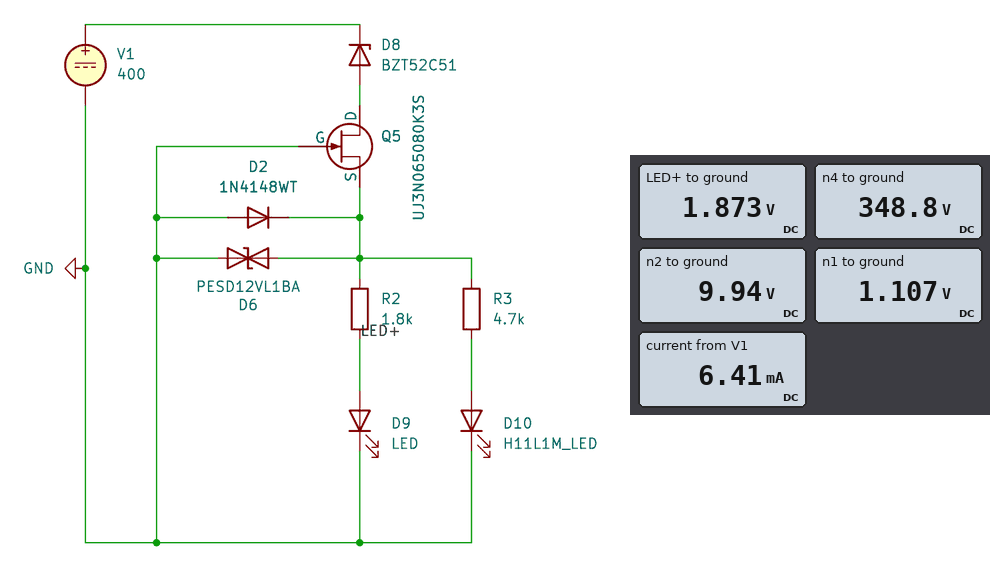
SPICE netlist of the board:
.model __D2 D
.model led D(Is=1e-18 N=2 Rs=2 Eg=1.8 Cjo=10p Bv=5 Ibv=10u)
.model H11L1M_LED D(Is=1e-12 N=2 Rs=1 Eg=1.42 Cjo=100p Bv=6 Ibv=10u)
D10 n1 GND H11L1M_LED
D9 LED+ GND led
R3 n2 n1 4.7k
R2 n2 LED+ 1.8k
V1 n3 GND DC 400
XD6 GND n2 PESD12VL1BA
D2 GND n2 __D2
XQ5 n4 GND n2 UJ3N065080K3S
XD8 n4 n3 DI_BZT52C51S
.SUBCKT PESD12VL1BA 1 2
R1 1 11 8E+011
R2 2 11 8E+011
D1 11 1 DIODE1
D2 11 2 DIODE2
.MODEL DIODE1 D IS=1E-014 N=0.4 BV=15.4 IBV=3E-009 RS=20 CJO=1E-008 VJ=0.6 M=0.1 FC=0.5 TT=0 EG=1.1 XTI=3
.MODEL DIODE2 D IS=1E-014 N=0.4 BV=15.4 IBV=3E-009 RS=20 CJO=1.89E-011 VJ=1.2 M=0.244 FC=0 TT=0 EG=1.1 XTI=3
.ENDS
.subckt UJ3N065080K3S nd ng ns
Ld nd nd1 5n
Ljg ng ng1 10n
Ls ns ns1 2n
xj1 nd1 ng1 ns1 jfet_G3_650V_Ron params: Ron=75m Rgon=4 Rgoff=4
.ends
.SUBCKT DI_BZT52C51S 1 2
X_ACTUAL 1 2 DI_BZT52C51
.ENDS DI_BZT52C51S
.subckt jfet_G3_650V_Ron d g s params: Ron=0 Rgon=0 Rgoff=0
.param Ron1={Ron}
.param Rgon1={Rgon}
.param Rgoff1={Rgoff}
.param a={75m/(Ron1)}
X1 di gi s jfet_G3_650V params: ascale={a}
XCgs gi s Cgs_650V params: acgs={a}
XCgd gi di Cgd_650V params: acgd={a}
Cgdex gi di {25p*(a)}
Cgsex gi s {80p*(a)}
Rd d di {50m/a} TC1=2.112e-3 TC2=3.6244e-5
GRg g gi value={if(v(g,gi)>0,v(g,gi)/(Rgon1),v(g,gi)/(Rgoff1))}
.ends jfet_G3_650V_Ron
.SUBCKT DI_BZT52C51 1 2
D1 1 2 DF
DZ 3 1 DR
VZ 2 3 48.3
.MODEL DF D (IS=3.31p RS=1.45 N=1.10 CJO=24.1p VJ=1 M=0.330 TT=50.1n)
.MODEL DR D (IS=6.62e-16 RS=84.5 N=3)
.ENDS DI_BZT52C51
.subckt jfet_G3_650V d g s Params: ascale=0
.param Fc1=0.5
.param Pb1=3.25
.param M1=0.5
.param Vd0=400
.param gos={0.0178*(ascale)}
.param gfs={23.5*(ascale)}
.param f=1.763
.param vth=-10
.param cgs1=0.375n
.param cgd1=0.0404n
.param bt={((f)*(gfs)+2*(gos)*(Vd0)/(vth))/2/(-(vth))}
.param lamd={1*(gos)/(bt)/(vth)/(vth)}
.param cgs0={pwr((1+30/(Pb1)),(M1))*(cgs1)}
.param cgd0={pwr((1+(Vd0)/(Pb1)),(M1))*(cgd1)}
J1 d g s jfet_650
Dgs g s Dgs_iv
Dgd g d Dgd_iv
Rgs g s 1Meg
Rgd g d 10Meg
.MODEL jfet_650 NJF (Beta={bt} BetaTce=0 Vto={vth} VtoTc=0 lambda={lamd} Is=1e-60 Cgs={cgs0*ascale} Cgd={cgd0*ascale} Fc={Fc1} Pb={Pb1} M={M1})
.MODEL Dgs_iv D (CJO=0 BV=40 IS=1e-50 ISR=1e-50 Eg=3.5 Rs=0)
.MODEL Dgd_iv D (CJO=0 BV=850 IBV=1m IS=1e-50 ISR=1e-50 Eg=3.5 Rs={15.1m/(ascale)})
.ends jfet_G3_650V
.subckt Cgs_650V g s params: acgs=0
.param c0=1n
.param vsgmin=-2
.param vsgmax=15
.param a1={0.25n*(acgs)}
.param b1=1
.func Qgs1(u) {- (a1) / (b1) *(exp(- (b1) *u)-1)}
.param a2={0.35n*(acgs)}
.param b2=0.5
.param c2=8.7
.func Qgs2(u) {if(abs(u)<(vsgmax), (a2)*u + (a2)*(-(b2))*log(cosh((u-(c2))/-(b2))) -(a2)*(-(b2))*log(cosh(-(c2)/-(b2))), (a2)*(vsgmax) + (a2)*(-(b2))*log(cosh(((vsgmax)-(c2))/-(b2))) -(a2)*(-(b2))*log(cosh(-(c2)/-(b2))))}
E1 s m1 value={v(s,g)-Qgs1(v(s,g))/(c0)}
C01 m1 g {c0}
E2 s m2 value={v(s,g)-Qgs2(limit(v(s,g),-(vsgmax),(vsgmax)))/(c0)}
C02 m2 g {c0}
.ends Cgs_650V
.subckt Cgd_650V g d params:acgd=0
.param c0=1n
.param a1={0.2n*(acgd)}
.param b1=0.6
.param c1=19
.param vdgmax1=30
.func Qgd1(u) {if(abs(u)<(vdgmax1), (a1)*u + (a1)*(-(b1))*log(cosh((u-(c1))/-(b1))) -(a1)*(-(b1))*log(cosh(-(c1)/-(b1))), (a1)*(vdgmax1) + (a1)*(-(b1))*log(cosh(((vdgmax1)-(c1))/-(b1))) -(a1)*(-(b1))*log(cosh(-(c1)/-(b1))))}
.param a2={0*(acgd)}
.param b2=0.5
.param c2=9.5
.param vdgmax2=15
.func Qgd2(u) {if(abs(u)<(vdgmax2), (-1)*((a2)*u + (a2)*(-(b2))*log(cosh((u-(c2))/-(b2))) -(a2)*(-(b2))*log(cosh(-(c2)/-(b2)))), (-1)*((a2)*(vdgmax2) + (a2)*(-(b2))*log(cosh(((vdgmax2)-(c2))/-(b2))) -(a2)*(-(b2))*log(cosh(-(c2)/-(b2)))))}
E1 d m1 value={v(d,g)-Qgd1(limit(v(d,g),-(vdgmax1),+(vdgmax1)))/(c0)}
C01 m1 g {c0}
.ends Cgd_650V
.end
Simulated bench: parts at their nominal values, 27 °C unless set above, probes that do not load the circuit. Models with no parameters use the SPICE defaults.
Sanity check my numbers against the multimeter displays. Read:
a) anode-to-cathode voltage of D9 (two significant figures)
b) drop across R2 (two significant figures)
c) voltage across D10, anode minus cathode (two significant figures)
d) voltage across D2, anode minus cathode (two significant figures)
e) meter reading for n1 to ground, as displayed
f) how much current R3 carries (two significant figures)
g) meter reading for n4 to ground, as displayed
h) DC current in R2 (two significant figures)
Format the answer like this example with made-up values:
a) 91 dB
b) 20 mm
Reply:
a) 1.9 V
b) 8.1 V
c) 1.1 V
d) -9.9 V
e) 1.107 V
f) 1.9 mA
g) 348.8 V
h) 4.5 mA
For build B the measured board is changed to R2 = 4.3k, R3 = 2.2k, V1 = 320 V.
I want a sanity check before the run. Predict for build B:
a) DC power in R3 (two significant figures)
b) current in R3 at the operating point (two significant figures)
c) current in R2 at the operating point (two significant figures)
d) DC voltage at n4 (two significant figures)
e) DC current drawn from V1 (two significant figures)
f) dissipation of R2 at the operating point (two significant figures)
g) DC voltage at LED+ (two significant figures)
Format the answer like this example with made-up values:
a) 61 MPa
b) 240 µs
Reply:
a) 35 mW
b) 4.0 mA
c) 1.9 mA
d) 270 V
e) 5.9 mA
f) 15 mW
g) 1.8 V
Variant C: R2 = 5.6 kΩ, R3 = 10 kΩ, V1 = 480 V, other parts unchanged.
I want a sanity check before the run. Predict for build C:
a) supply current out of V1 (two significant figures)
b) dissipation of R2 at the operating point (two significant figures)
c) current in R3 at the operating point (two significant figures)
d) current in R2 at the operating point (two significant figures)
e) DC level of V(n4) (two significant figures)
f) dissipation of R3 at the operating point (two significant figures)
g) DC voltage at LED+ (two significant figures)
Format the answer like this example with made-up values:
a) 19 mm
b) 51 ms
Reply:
a) 2.4 mA
b) 12 mW
c) 890 µA
d) 1.5 mA
e) 430 V
f) 7.9 mW
g) 1.8 V
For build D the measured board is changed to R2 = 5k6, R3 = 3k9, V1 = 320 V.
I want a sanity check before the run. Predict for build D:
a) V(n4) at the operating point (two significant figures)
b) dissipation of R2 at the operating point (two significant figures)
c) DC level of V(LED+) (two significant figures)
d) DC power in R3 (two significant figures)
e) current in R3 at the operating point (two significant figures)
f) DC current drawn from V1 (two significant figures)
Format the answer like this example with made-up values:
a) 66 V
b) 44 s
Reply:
a) 270 V
b) 12 mW
c) 1.8 V
d) 20 mW
e) 2.3 mA
f) 3.8 mA
